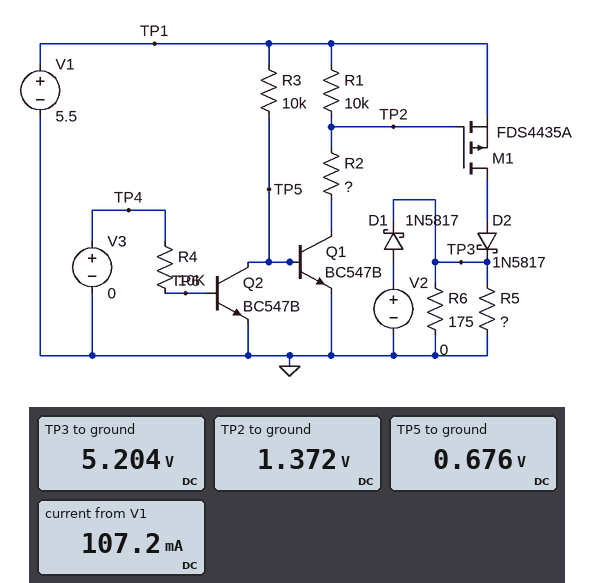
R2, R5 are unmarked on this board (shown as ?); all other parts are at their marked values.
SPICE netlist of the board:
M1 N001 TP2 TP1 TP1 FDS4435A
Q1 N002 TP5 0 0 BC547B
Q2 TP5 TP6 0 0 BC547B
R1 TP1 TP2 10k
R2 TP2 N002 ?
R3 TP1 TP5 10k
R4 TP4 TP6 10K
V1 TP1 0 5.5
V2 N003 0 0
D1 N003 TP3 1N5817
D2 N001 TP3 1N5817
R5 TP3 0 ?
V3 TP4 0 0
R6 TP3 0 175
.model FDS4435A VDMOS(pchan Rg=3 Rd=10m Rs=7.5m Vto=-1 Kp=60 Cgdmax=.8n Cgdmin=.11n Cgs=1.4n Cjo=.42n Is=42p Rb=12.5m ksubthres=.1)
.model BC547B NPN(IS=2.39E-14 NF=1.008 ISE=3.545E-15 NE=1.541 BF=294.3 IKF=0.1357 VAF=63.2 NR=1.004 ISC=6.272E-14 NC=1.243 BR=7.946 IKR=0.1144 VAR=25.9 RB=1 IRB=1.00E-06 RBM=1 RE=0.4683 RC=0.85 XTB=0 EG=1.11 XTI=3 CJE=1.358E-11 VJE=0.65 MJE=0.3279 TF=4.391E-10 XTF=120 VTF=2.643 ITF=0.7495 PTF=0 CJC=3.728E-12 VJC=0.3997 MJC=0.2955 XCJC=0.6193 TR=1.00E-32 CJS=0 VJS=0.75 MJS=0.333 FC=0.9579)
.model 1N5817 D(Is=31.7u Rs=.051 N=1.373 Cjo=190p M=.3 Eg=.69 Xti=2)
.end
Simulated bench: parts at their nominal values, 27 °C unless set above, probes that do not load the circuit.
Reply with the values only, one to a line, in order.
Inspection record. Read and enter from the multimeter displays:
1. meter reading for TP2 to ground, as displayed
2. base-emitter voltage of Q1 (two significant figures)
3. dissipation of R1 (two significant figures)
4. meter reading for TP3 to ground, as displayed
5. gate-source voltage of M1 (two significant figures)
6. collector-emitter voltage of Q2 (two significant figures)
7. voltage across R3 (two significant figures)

1.372 V
680 mV
1.7 mW
5.204 V
-4.1 V
680 mV
4.8 V
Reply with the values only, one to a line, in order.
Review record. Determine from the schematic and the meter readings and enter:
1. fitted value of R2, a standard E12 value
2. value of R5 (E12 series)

3.3 kΩ
68 Ω
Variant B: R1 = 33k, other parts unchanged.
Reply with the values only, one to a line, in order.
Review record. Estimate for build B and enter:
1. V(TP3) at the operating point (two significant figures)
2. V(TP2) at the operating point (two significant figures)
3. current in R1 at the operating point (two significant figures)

5.2 V
510 mV
150 µA
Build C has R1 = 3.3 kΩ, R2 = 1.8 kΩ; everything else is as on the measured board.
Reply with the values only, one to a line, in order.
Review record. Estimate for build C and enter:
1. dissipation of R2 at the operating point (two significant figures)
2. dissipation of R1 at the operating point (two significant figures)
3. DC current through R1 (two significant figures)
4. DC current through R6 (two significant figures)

2.1 mW
3.8 mW
1.1 mA
30 mA
